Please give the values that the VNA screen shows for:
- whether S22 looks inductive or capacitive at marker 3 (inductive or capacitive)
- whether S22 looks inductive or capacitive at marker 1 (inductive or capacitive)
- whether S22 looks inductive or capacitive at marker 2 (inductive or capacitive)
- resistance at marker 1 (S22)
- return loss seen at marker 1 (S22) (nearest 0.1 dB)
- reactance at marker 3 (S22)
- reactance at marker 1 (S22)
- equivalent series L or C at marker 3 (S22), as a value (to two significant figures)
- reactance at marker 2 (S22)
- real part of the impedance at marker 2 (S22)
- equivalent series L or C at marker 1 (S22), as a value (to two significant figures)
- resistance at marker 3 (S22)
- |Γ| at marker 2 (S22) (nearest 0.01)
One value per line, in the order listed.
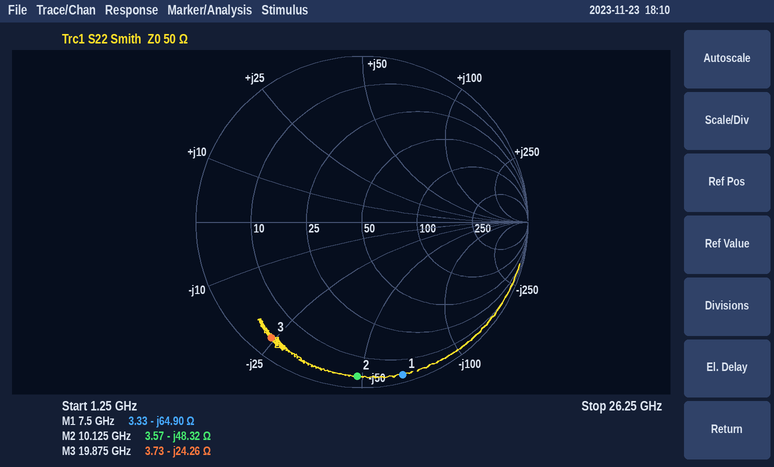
capacitive
capacitive
capacitive
3.33 Ω
0.4 dB
-24.26 Ω
-64.90 Ω
330 fF
-48.32 Ω
3.57 Ω
330 fF
3.73 Ω
0.93
